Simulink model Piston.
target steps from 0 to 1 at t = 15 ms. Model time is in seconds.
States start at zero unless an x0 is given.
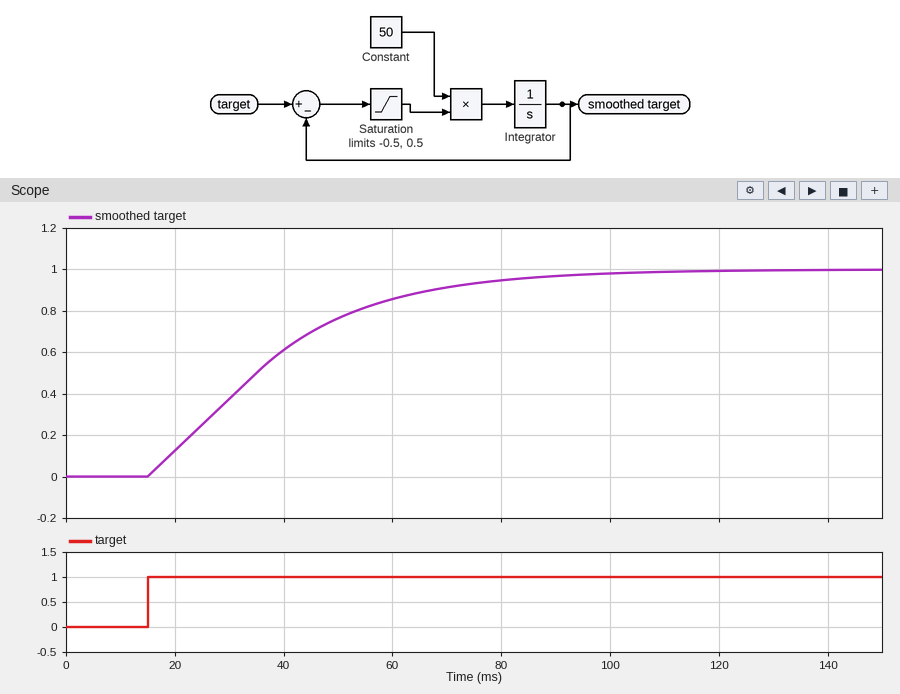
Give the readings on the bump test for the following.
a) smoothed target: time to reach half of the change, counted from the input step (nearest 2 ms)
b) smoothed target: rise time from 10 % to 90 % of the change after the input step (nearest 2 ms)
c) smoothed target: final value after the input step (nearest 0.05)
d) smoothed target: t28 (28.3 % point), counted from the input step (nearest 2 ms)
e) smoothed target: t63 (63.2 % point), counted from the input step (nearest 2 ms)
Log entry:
20 ms
48 ms
1.00
12 ms
26 ms
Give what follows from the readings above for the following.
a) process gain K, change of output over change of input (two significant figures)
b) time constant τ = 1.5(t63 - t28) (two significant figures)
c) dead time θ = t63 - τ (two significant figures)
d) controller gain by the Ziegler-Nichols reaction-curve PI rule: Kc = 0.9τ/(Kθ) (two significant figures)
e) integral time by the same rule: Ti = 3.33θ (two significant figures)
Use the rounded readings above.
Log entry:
1.0
21 ms
5.0 ms
3.8
17 ms
